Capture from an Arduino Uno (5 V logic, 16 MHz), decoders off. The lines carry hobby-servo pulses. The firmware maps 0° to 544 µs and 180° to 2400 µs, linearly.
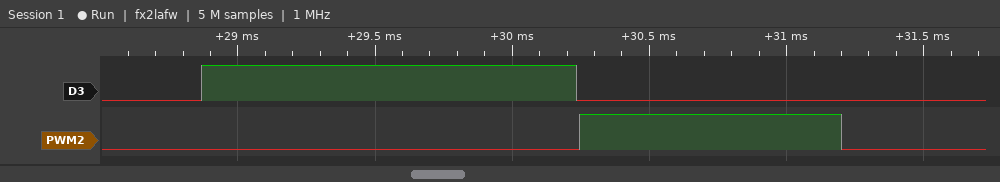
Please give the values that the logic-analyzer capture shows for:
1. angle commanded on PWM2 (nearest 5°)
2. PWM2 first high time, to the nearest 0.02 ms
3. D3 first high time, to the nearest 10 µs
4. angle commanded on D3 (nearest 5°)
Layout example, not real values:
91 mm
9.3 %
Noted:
40°
0.96 ms
1370 µs
80°
